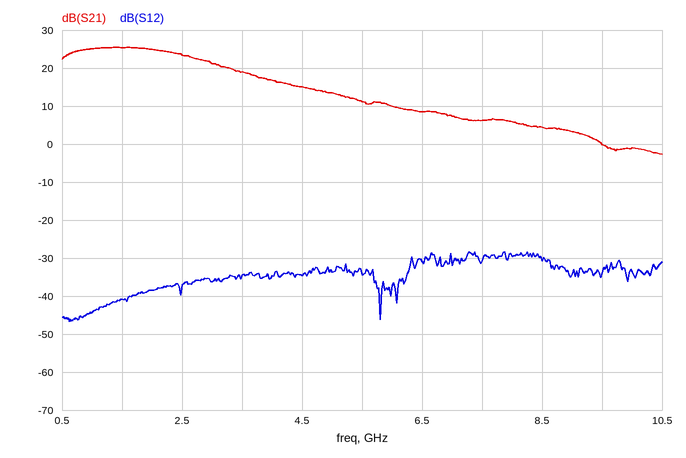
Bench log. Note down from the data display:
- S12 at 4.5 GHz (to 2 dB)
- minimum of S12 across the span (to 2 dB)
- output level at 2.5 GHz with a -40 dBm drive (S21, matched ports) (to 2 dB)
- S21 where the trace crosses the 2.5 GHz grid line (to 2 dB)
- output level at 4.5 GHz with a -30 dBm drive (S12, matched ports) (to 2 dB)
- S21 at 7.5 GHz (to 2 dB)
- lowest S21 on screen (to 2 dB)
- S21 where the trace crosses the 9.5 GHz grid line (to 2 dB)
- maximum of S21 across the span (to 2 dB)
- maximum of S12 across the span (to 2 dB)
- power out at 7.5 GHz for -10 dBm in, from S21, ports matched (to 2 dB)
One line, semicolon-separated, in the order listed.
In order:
-34 dB; -46 dB; -16 dBm; 24 dB; -64 dBm; 6 dB; -2 dB; 0 dB; 26 dB; -28 dB; -4 dBm
